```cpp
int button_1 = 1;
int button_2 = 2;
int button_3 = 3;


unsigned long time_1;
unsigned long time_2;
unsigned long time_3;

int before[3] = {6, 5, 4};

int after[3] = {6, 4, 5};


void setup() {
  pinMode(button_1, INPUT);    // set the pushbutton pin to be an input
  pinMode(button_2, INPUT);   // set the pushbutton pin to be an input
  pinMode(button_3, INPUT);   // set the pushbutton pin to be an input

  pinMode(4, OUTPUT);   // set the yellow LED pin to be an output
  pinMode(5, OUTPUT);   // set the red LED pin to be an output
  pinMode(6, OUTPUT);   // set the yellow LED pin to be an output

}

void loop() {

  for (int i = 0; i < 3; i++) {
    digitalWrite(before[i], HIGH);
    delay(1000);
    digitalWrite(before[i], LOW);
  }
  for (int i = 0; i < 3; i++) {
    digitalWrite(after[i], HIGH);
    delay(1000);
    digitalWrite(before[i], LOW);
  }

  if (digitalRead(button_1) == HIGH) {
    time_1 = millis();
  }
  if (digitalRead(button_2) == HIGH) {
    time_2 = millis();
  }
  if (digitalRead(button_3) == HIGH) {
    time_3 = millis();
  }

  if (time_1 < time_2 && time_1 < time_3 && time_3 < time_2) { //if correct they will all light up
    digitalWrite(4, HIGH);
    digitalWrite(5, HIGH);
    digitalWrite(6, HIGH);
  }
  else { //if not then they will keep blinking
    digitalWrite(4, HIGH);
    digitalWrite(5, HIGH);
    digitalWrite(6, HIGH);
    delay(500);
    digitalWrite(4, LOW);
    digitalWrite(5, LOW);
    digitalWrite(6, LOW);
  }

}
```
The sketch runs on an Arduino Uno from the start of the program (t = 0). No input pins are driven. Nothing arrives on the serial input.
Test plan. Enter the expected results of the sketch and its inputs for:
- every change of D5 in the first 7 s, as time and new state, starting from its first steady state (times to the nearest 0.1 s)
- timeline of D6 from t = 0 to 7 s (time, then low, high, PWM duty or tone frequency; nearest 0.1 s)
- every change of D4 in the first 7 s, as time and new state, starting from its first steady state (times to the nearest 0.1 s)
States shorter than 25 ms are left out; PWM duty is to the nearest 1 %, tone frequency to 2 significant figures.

0 s low; 1 s high; 2 s low; 5 s high; 6.5 s low
0 s high; 1 s low; 3 s high; 4 s low; 6 s high
0 s low; 2 s high; 3 s low; 4 s high; 6.5 s low
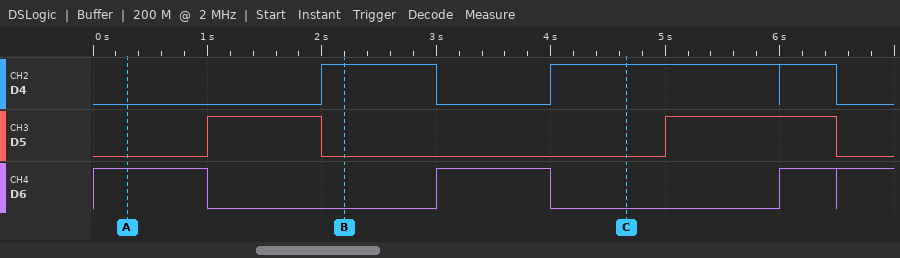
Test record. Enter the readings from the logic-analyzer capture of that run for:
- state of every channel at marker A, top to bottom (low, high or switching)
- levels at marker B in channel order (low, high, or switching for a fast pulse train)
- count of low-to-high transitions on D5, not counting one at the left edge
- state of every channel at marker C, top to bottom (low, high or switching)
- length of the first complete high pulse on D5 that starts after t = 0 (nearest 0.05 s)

D4 low, D5 low, D6 high
D4 high, D5 low, D6 low
2
D4 high, D5 low, D6 low
1.00 s
